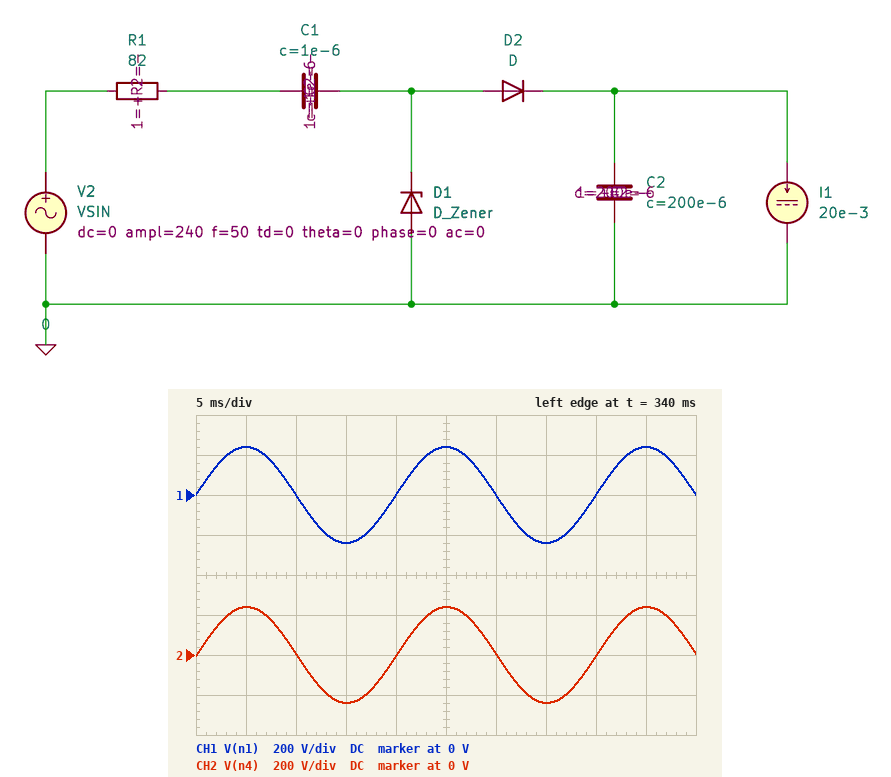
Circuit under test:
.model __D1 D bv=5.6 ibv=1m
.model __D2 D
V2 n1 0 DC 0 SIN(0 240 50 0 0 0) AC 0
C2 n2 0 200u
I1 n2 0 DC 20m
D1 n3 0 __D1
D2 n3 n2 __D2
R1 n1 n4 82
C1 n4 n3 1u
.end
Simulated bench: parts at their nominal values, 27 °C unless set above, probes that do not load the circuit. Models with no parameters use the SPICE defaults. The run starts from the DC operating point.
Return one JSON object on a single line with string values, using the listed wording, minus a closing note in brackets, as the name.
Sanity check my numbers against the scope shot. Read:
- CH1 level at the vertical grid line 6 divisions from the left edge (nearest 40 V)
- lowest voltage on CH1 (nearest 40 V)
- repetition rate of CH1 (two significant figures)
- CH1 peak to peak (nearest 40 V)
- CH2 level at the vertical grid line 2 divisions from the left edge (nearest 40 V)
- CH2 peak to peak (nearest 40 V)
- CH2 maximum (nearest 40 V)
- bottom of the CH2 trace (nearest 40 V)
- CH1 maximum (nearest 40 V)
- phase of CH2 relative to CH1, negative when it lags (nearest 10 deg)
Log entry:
{"CH1 level at the vertical grid line 6 divisions from the left edge": "0 V", "lowest voltage on CH1": "-240 V", "repetition rate of CH1": "50 Hz", "CH1 peak to peak": "480 V", "CH2 level at the vertical grid line 2 divisions from the left edge": "0 V", "CH2 peak to peak": "480 V", "CH2 maximum": "240 V", "bottom of the CH2 trace": "-240 V", "CH1 maximum": "240 V", "phase of CH2 relative to CH1, negative when it lags": "0 deg"}
